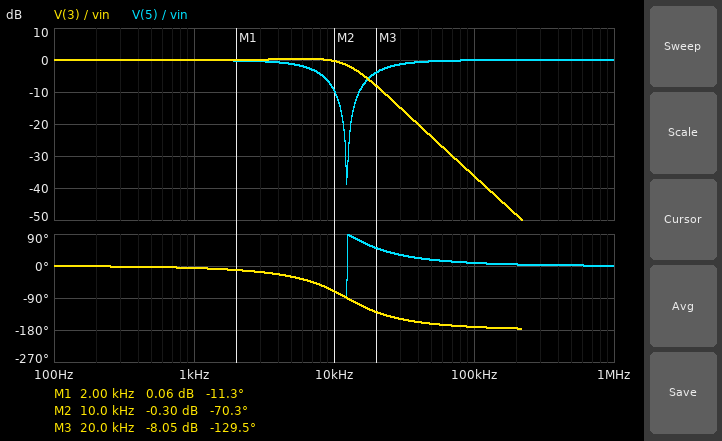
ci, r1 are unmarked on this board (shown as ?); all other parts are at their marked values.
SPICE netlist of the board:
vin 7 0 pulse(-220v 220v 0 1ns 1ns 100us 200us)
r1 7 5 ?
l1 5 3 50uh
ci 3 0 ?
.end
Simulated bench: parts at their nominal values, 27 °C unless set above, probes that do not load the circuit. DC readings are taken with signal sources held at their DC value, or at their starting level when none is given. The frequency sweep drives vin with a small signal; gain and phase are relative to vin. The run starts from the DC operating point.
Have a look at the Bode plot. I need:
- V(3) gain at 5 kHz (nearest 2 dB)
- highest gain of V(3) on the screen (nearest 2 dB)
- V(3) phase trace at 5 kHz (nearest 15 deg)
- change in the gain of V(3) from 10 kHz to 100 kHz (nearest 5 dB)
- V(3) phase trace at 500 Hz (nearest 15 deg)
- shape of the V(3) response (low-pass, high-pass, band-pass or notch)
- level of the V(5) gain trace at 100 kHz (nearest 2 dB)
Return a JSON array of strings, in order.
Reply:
["0 dB", "0 dB", "-30 deg", "-35 dB", "0 deg", "low-pass", "0 dB"]
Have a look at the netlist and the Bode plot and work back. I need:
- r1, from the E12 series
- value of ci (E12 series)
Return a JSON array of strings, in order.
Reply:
["4.7 Ω", "3.3 µF"]
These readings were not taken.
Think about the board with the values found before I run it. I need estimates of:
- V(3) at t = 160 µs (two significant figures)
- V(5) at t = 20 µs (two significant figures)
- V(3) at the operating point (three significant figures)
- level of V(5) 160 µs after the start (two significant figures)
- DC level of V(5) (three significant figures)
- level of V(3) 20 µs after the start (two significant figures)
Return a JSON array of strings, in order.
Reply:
["-250 V", "-26 V", "-220 V", "-240 V", "-220 V", "41 V"]
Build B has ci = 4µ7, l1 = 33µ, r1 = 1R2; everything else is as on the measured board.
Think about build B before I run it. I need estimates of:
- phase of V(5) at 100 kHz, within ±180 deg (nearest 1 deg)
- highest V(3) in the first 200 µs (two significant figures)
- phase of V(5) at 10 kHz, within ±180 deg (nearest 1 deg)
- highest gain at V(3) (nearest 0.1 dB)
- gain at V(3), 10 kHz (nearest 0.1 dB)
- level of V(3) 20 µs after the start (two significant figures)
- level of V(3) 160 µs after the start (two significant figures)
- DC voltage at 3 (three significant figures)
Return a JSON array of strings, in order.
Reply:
["3 deg", "430 V", "-42 deg", "7.1 dB", "5.6 dB", "150 V", "-280 V", "-220 V"]
